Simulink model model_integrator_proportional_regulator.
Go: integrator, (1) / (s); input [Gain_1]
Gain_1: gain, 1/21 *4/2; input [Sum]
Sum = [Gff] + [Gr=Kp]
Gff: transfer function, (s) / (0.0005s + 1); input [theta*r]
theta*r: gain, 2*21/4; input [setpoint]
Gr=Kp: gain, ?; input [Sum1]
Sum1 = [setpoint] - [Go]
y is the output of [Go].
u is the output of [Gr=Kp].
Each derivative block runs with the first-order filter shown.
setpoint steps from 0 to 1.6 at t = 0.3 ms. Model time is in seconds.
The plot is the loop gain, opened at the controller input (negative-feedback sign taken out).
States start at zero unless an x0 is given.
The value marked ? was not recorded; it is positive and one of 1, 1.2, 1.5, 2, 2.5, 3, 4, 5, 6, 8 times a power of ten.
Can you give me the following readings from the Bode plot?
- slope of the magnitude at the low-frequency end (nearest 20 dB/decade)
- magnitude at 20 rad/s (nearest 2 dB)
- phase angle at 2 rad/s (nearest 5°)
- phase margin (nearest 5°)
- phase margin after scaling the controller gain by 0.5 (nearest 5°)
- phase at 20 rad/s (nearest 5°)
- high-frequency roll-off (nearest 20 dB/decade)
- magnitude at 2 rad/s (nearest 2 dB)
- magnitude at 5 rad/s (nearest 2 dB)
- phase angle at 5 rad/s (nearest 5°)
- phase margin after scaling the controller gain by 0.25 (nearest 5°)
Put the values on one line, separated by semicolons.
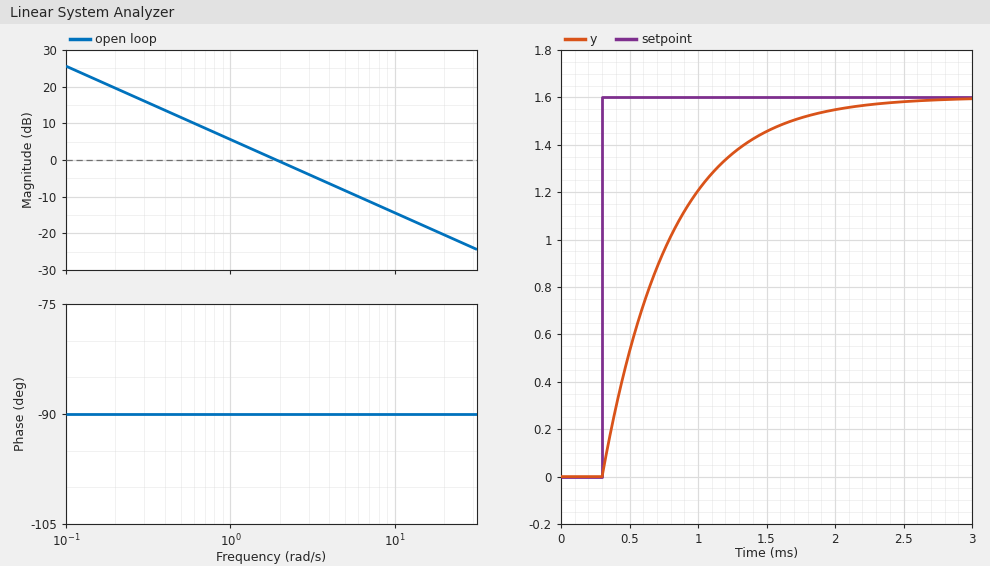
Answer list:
-20 dB/decade; -20 dB; -90°; 90°; 90°; -90°; -20 dB/decade; 0 dB; -8 dB; -90°; 90°
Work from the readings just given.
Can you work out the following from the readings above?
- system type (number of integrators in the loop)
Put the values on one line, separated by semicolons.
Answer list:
1
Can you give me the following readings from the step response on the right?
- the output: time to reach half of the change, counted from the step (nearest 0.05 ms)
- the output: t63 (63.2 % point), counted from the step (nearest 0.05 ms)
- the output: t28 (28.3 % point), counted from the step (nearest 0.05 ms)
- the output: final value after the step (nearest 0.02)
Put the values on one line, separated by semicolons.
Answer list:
0.35 ms; 0.50 ms; 0.15 ms; 1.60
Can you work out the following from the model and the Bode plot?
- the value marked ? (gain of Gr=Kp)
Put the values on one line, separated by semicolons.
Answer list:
20
